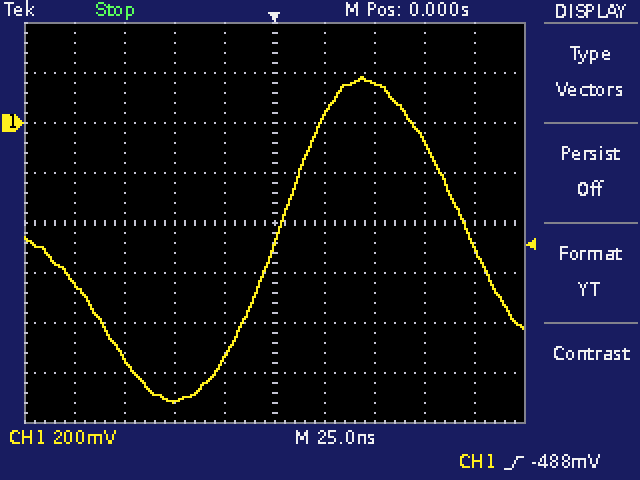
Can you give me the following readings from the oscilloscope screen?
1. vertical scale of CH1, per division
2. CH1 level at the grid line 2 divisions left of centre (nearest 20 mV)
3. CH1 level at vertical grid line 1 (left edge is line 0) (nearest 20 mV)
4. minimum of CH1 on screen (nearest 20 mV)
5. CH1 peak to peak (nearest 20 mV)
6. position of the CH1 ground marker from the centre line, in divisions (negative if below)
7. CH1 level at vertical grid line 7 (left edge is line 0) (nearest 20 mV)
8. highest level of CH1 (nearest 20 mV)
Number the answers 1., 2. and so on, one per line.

1. 200 mV
2. -1.12 V
3. -640 mV
4. -1.12 V
5. 1.30 V
6. +2.0 div
7. 160 mV
8. 180 mV
